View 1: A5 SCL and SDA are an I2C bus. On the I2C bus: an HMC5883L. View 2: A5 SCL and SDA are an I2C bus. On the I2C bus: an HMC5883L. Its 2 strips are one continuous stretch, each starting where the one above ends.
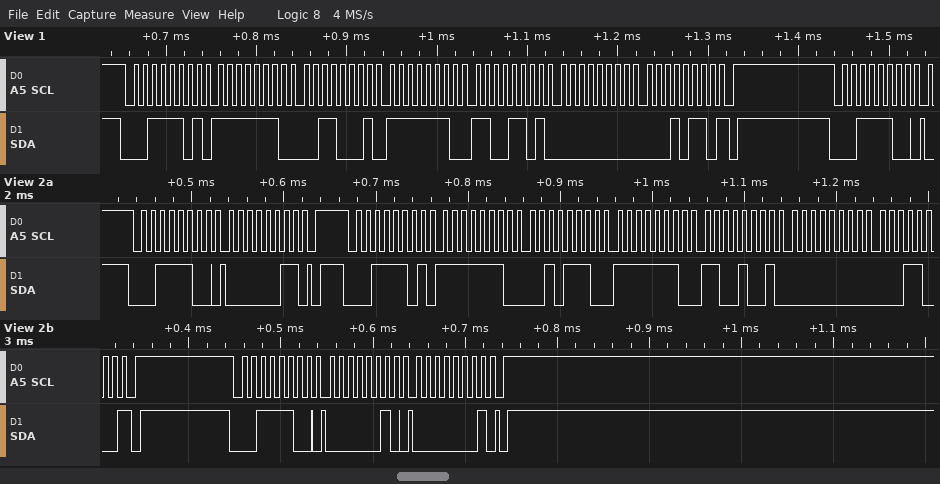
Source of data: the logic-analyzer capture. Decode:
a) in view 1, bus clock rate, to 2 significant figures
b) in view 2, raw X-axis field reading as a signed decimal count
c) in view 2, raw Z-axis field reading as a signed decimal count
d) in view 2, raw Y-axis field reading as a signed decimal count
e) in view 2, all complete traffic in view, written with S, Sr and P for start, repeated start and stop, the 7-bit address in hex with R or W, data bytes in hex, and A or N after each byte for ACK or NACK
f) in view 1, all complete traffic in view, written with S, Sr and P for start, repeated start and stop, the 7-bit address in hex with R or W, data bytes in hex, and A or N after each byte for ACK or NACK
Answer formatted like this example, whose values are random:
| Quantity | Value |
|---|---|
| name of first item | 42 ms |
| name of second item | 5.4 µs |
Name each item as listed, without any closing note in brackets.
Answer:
| Quantity | Value |
|---|---|
| in view 1, bus clock rate, to 2 significant figures | 100 kHz |
| in view 2, raw X-axis field reading as a signed decimal count | -466 |
| in view 2, raw Z-axis field reading as a signed decimal count | -311 |
| in view 2, raw Y-axis field reading as a signed decimal count | 24 |
| in view 2, all complete traffic in view, written with S, Sr and P for start, repeated start and stop, the 7-bit address in hex with R or W, data bytes in hex, and A or N after each byte for ACK or NACK | S 1EW A 03 A P S 1ER A FE A 2E A FE A C9 A 00 A 18 N P S 1EW A 02 A 01 A P |
| in view 1, all complete traffic in view, written with S, Sr and P for start, repeated start and stop, the 7-bit address in hex with R or W, data bytes in hex, and A or N after each byte for ACK or NACK | S 1ER A FE A 31 A FE A CD A 00 A 16 N P S 1EW A |
